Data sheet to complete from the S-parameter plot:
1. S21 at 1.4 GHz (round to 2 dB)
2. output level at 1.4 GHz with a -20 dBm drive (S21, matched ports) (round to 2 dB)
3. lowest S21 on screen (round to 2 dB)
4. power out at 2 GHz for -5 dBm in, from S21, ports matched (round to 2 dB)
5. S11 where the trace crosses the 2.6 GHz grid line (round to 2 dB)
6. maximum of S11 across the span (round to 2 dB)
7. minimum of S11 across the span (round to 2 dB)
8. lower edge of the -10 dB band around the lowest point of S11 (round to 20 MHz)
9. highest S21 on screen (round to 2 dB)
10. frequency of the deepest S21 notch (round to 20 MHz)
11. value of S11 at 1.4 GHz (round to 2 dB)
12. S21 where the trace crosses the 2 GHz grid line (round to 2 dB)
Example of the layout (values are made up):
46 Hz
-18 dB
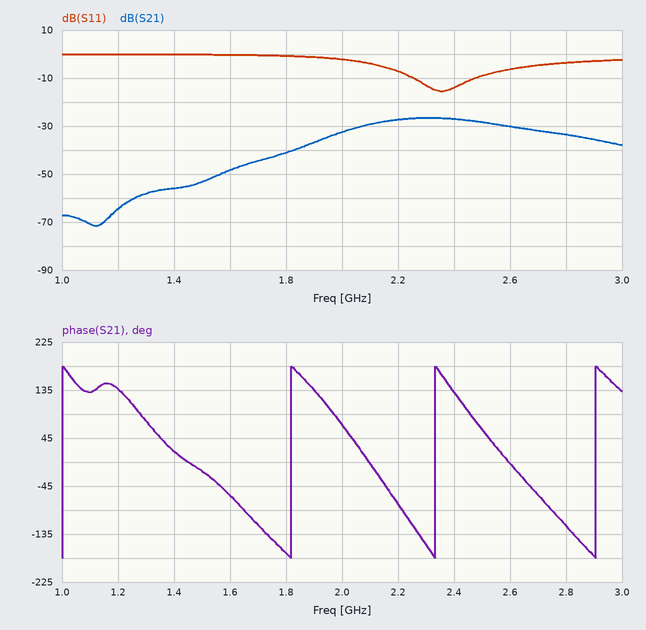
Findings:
-56 dB
-76 dBm
-72 dB
-38 dBm
-6 dB
0 dB
-16 dB
2.26 GHz
-26 dB
1.12 GHz
0 dB
-32 dB
